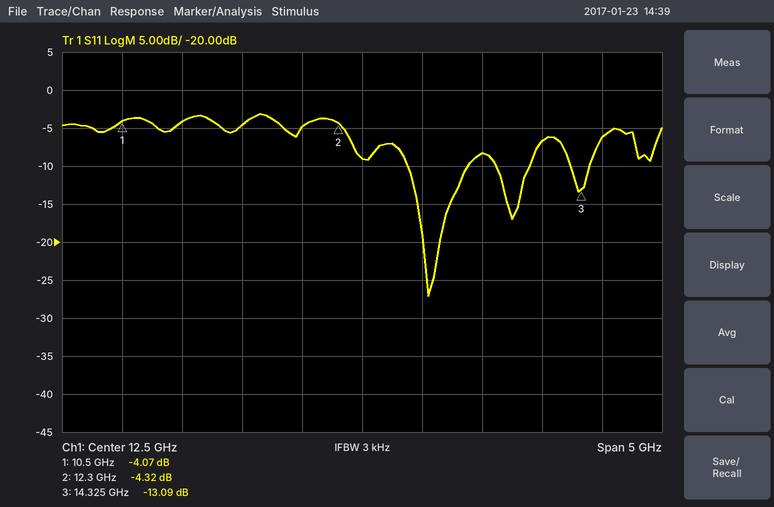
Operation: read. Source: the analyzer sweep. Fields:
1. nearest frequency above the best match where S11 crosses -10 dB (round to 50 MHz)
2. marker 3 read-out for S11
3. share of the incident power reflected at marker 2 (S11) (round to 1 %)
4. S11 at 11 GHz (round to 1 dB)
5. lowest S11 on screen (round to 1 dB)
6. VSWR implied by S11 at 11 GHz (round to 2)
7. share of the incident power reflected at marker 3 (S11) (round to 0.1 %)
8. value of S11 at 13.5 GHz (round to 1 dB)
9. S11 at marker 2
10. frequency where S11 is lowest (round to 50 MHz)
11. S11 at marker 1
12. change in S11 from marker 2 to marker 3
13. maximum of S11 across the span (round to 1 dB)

13.40 GHz
-13.09 dB
37 %
-4 dB
-27 dB
4
4.9 %
-8 dB
-4.32 dB
13.05 GHz
-4.07 dB
-8.77 dB
-3 dB
